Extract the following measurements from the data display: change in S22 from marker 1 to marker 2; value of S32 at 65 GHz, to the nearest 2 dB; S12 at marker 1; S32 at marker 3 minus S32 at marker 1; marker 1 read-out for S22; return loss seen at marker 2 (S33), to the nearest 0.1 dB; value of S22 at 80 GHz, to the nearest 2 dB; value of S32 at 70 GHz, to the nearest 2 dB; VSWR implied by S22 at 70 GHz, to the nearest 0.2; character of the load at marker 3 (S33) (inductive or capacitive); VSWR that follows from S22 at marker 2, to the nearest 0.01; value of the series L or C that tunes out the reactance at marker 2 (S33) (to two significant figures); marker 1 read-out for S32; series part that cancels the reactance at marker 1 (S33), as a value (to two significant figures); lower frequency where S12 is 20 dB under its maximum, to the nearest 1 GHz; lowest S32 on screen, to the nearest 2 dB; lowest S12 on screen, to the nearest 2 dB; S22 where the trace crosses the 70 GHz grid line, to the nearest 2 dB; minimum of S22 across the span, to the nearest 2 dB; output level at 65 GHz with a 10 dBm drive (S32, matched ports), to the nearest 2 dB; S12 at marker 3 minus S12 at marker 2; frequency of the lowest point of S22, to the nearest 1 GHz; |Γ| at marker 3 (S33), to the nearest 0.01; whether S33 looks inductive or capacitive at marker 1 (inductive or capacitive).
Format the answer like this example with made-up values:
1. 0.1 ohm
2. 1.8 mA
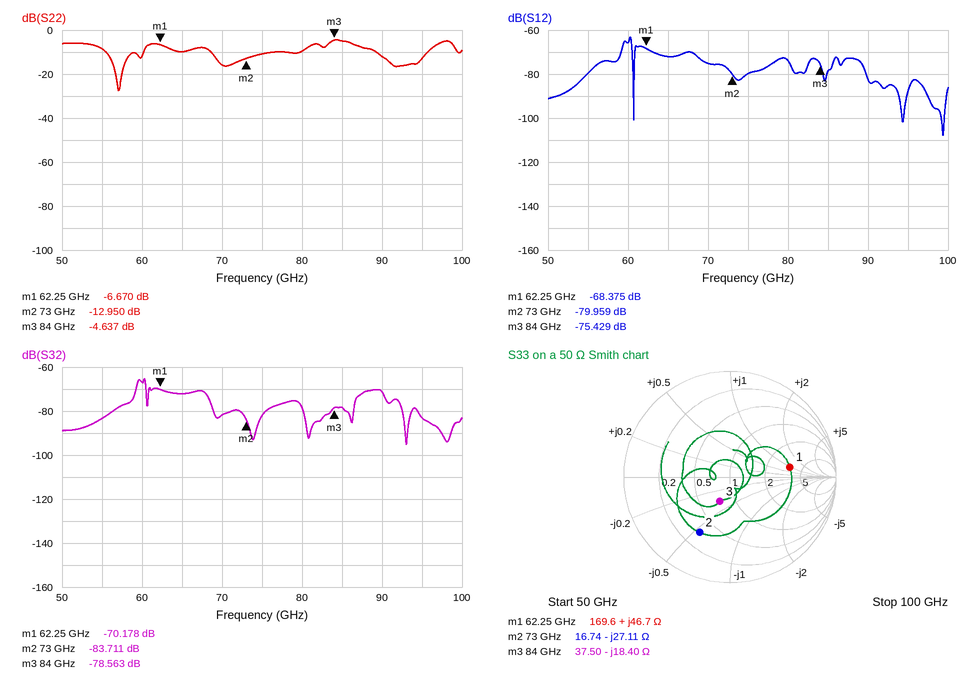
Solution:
1. -6.280 dB
2. -72 dB
3. -68.375 dB
4. -8.385 dB
5. -6.670 dB
6. 4.5 dB
7. -10 dB
8. -82 dB
9. 1.4
10. capacitive
11. 1.58
12. 59 pH
13. -70.178 dB
14. 55 fF
15. 54 GHz
16. -96 dB
17. -108 dB
18. -16 dB
19. -28 dB
20. -62 dBm
21. 4.530 dB
22. 57 GHz
23. 0.25
24. inductive
